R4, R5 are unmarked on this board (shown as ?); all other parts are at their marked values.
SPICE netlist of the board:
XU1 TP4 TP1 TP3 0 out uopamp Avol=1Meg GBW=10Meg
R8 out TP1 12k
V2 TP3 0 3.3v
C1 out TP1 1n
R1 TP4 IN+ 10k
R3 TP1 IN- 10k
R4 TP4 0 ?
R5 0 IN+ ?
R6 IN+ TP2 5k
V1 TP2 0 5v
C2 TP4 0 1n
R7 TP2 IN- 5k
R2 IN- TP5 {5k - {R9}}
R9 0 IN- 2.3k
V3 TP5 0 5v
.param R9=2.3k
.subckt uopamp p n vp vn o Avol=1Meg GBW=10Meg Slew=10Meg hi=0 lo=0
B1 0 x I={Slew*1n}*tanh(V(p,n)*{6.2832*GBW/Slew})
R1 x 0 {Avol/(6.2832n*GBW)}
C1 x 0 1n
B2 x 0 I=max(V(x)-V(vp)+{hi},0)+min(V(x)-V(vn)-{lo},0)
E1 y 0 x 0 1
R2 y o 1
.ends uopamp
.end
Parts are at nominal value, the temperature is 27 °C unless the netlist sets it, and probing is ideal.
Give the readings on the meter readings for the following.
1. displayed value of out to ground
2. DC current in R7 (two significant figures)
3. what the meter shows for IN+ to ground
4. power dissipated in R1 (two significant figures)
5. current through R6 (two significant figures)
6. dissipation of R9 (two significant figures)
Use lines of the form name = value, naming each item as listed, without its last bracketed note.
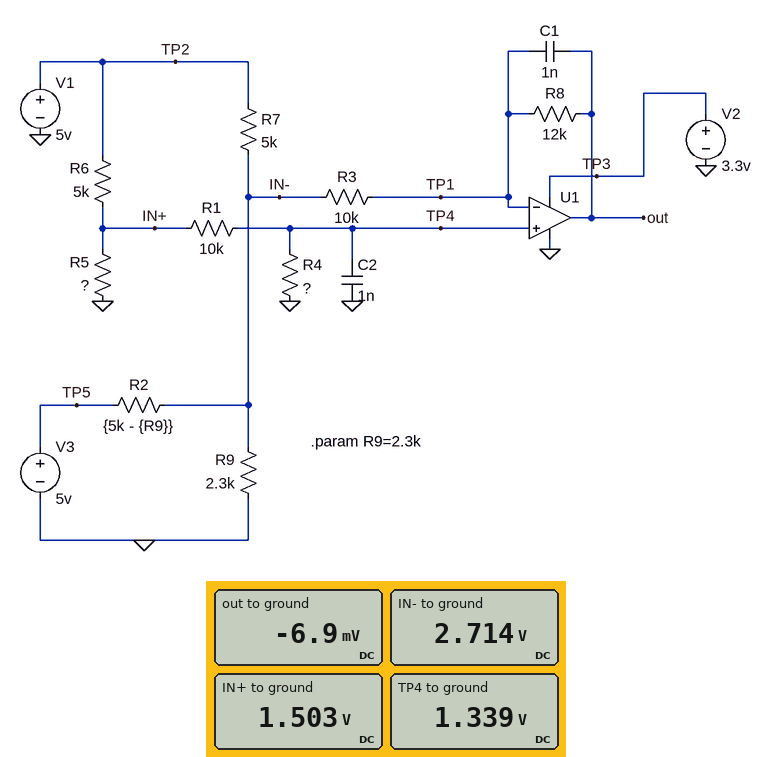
displayed value of out to ground = -6.9 mV
DC current in R7 = 460 µA
what the meter shows for IN+ to ground = 1.503 V
power dissipated in R1 = 2.7 µW
current through R6 = 700 µA
dissipation of R9 = 3.2 mW
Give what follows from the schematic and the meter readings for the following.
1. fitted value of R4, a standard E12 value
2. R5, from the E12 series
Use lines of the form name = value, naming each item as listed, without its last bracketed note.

fitted value of R4, a standard E12 value = 82 kΩ
R5, from the E12 series = 2.2 kΩ
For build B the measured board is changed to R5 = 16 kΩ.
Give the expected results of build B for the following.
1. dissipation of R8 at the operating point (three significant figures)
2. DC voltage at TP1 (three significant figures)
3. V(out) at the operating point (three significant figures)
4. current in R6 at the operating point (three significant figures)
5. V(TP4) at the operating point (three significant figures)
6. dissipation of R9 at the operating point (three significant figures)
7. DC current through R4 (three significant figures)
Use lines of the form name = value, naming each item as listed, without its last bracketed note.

dissipation of R8 at the operating point = 5.04 µW
DC voltage at TP1 = 3.06 V
V(out) at the operating point = 3.31 V
current in R6 at the operating point = 268 µA
V(TP4) at the operating point = 3.26 V
dissipation of R9 at the operating point = 3.55 mW
DC current through R4 = 39.8 µA
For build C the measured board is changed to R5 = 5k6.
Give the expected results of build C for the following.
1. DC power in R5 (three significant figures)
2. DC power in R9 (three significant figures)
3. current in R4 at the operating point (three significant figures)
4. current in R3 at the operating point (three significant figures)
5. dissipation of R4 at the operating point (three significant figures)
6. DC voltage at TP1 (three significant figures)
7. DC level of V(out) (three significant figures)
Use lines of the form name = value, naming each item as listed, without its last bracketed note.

DC power in R5 = 1.18 mW
DC power in R9 = 3.38 mW
current in R4 at the operating point = 27.9 µA
current in R3 at the operating point = 49.9 µA
dissipation of R4 at the operating point = 63.9 µW
DC voltage at TP1 = 2.29 V
DC level of V(out) = 1.69 V
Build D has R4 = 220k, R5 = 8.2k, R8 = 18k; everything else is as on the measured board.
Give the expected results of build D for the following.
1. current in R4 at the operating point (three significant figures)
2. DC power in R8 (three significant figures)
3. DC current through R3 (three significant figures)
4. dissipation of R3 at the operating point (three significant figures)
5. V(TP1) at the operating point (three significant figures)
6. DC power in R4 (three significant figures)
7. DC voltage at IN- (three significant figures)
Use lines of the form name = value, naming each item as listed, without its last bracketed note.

current in R4 at the operating point = 13.3 µA
DC power in R8 = 1.32 µW
DC current through R3 = 8.57 µA
dissipation of R3 at the operating point = 734 nW
V(TP1) at the operating point = 2.93 V
DC power in R4 = 39.1 µW
DC voltage at IN- = 2.85 V
